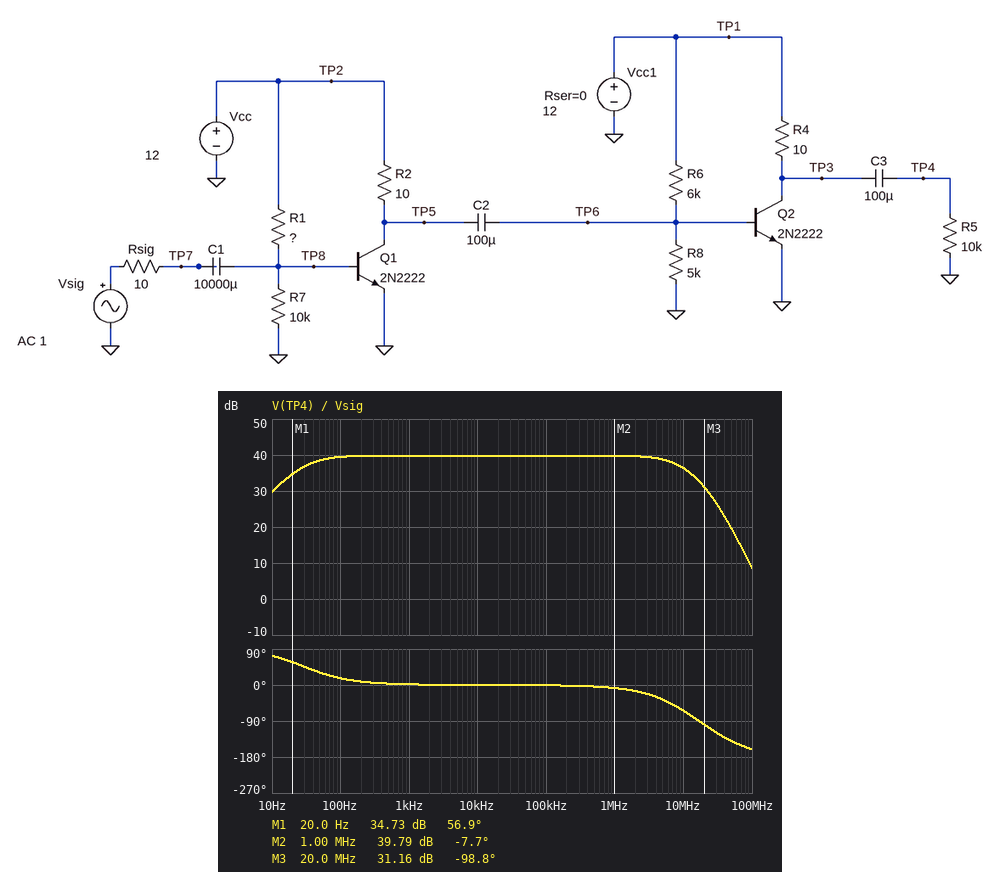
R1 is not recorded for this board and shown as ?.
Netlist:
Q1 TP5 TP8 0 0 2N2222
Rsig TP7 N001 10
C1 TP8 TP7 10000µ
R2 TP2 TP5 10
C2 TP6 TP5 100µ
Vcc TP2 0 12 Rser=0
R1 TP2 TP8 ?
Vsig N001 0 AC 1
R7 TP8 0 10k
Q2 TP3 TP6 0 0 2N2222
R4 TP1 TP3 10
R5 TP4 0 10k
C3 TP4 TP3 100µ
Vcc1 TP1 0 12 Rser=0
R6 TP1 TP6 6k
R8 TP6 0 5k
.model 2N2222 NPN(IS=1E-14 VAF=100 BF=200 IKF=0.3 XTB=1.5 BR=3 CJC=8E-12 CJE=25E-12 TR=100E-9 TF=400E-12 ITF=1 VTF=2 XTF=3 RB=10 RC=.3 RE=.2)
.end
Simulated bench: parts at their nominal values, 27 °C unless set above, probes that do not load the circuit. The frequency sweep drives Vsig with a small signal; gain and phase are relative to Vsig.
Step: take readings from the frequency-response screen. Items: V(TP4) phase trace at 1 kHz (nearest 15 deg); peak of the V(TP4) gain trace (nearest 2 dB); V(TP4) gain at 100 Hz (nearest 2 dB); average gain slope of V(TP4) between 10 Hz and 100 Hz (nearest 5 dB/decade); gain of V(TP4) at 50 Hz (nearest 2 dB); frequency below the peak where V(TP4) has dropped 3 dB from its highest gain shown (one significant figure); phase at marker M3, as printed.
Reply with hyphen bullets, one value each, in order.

- 0 deg
- 40 dB
- 40 dB
- 10 dB/decade
- 38 dB
- 30 Hz
- -98.8 deg
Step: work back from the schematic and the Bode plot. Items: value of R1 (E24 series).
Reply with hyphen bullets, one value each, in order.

- 68 kΩ
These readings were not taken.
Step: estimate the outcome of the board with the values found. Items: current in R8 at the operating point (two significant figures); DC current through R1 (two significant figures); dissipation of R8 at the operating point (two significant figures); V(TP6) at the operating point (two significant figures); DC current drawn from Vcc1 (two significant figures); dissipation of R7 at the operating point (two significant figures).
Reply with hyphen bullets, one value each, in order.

- 170 µA
- 170 µA
- 150 µW
- 870 mV
- 220 mA
- 54 µW
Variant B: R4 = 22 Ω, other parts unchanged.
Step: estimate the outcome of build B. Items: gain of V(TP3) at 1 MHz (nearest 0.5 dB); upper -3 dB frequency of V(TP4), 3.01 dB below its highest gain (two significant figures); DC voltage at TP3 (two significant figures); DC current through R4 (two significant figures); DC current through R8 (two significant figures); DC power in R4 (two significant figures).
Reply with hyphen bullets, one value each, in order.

- 46.5 dB
- 8.2 MHz
- 7.3 V
- 210 mA
- 170 µA
- 1.0 W
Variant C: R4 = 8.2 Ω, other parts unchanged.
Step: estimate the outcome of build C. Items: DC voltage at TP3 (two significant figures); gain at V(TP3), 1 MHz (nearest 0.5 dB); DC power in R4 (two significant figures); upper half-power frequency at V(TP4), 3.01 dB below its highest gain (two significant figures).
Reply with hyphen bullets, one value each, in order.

- 10 V
- 38.0 dB
- 400 mW
- 9.2 MHz
